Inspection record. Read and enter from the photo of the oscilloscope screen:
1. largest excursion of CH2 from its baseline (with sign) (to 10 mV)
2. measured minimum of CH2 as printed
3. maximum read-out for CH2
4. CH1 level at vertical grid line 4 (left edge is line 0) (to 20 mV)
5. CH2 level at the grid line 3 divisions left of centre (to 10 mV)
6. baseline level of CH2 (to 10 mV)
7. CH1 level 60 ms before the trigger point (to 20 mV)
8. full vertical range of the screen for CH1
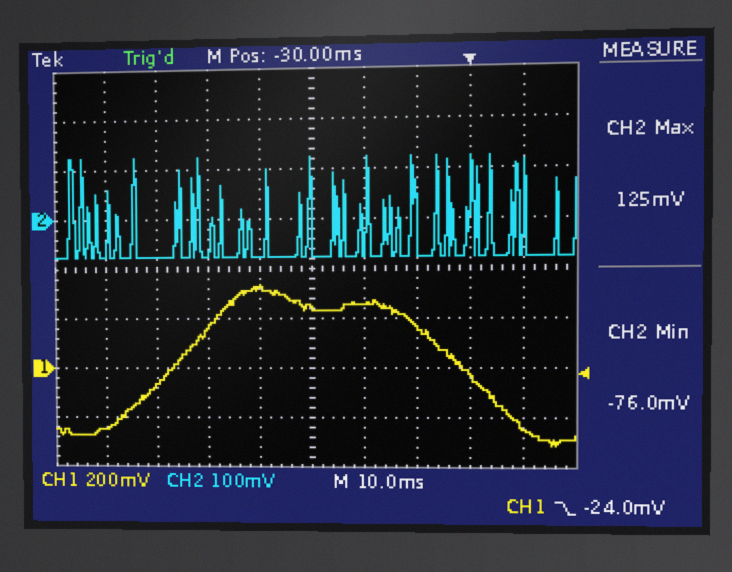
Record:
+200 mV
-76.0 mV
125 mV
320 mV
-80 mV
-80 mV
-60 mV
1.6 V
